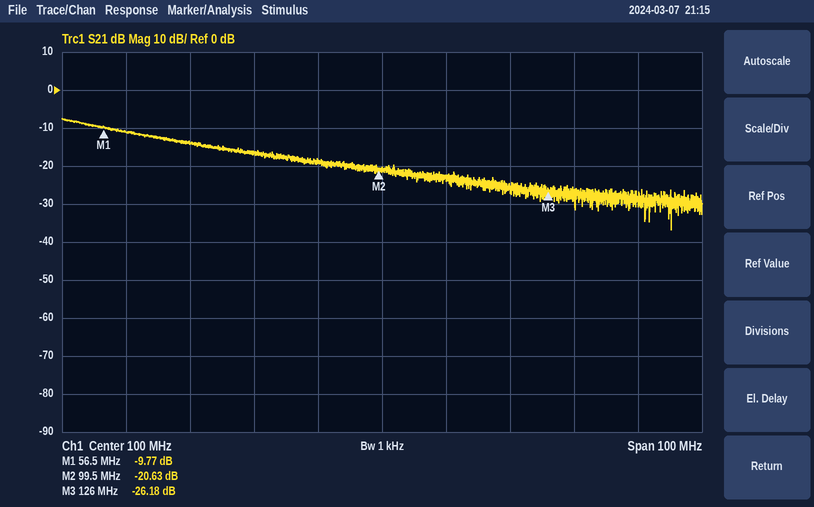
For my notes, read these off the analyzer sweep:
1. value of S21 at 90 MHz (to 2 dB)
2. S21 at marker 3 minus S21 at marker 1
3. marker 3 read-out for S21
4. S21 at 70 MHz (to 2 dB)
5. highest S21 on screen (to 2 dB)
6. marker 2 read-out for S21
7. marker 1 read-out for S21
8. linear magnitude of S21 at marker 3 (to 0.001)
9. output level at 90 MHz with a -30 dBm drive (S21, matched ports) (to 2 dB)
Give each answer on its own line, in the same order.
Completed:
-18 dB
-16.41 dB
-26.18 dB
-14 dB
-8 dB
-20.63 dB
-9.77 dB
0.049
-48 dBm
